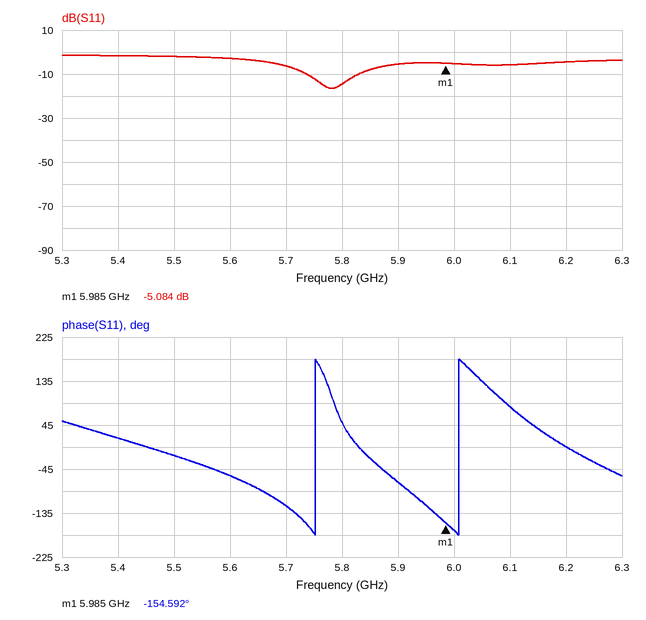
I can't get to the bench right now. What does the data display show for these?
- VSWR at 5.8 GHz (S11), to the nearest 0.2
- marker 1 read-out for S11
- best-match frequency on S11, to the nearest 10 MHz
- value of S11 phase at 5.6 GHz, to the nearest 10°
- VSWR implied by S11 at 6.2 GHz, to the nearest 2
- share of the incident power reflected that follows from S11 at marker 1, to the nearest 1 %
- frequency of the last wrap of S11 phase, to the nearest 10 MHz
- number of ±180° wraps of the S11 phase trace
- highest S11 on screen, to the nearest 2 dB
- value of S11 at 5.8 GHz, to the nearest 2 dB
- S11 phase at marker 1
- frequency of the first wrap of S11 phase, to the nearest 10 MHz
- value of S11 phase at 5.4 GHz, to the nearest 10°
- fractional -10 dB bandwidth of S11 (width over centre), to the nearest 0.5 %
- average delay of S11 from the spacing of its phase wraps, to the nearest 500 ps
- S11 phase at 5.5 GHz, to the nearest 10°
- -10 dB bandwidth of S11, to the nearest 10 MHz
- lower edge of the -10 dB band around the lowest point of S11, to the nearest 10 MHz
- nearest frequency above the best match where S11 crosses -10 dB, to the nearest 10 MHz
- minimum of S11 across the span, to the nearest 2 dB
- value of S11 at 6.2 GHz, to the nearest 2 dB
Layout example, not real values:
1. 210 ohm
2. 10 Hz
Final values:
1. 1.4
2. -5.084 dB
3. 5.78 GHz
4. -60°
5. 4
6. 31 %
7. 6.01 GHz
8. 2
9. -2 dB
10. -14 dB
11. -154.592°
12. 5.75 GHz
13. 20°
14. 1.5 %
15. 4.0 ns
16. -20°
17. 90 MHz
18. 5.74 GHz
19. 5.83 GHz
20. -16 dB
21. -4 dB
